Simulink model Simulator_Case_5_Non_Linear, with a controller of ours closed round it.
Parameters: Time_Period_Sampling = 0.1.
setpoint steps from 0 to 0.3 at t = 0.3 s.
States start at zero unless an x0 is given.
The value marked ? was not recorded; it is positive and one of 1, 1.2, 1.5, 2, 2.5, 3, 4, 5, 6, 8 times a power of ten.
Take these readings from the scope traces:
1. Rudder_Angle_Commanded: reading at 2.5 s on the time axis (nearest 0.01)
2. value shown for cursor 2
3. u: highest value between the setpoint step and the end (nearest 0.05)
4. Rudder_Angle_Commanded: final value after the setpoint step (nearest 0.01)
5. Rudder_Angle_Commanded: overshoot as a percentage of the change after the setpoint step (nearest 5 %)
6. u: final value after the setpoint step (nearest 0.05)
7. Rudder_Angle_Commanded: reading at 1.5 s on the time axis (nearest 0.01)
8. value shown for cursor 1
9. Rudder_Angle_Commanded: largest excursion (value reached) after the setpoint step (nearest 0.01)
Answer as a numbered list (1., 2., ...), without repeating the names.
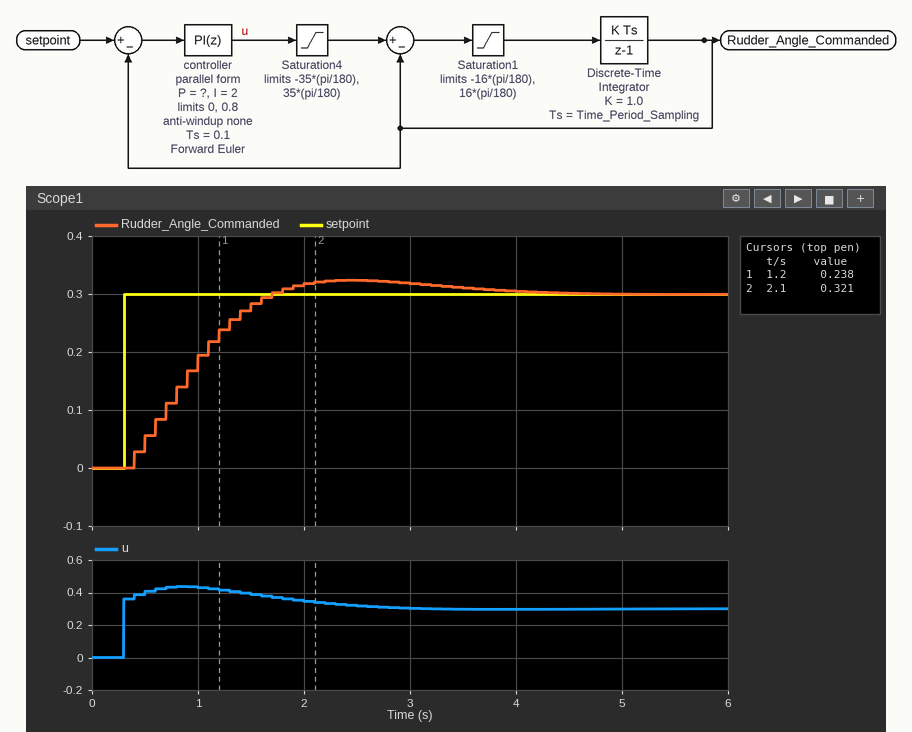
1. 0.32
2. 0.321
3. 0.45
4. 0.30
5. 10 %
6. 0.30
7. 0.28
8. 0.238
9. 0.32
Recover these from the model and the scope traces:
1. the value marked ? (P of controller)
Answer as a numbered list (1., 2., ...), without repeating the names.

1. 1.2
